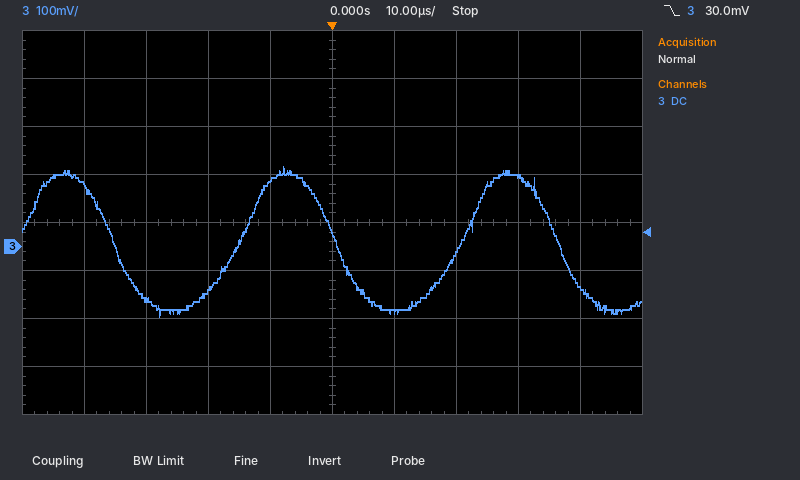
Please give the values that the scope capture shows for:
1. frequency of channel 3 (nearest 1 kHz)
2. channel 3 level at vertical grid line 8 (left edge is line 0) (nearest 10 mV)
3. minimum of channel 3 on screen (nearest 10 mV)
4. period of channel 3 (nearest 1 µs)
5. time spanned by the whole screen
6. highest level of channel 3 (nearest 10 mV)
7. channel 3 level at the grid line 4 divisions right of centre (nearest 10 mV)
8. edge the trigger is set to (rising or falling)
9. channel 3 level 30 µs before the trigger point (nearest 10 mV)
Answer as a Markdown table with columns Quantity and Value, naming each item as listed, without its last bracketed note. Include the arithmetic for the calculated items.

| Quantity | Value |
|---|---|
| frequency of channel 3 | 1 / 36 µs ≈ 28 kHz |
| channel 3 level at vertical grid line 8 (left edge is line 0) | 150 mV |
| minimum of channel 3 on screen | -150 mV |
| period of channel 3 | 36 µs |
| time spanned by the whole screen | 100 µs |
| highest level of channel 3 | 170 mV |
| channel 3 level at the grid line 4 divisions right of centre | -80 mV |
| edge the trigger is set to | falling |
| channel 3 level 30 µs before the trigger point | -110 mV |
